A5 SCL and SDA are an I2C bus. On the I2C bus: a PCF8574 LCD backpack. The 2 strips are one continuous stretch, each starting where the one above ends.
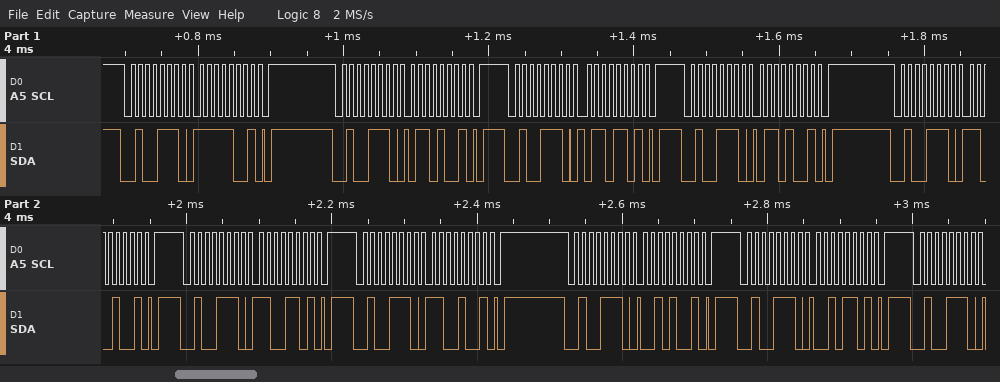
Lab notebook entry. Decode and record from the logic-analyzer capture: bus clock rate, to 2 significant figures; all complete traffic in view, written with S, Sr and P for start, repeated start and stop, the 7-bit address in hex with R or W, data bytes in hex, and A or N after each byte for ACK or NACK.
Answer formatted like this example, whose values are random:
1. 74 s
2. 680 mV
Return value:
1. 100 kHz
2. S 27W A F9 A P S 27W A 69 A P S 27W A 6D A P S 27W A 69 A P S 27W A C9 A P S 27W A CD A P S 27W A C9 A P S 27W A 29 A P S 27W A 2D A P S 27W A
